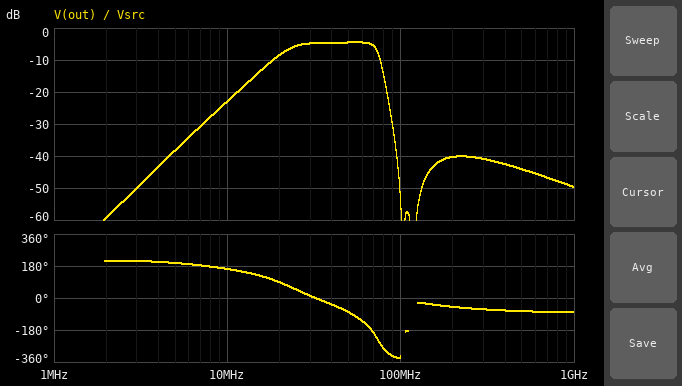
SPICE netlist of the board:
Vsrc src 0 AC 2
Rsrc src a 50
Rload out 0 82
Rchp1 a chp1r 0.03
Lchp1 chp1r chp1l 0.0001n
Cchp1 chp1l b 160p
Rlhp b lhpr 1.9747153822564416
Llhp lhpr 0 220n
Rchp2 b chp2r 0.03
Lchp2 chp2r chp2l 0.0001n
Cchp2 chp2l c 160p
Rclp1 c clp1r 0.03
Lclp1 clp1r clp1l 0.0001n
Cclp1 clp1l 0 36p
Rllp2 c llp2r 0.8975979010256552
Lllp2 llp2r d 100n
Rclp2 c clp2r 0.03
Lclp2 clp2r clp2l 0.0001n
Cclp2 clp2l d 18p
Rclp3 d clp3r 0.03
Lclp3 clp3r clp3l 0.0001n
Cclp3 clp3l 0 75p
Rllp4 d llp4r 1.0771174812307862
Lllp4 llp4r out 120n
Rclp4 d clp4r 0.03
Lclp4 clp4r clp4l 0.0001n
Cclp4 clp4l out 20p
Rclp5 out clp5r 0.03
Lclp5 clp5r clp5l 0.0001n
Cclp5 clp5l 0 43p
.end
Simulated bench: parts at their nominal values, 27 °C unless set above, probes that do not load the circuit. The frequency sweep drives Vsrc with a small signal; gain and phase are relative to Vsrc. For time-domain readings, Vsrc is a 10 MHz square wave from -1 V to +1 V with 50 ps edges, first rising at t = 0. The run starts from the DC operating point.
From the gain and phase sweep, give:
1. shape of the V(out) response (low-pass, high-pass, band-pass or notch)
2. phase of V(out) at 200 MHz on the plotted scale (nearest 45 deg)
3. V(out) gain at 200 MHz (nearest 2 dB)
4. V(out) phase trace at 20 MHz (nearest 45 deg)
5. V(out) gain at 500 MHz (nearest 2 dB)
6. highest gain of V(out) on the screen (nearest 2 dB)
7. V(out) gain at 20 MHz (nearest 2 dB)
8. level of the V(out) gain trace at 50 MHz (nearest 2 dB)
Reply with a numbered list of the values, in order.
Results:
1. band-pass
2. -45 deg
3. -40 dB
4. 90 deg
5. -44 dB
6. -4 dB
7. -8 dB
8. -4 dB
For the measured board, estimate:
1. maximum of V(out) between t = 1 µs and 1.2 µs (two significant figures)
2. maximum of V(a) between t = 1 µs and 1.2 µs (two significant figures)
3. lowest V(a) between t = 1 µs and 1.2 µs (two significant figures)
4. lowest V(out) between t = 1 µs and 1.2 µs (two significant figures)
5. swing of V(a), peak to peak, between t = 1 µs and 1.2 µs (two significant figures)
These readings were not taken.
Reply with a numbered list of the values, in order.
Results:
1. 490 mV
2. 1.2 V
3. -1.2 V
4. -490 mV
5. 2.4 V
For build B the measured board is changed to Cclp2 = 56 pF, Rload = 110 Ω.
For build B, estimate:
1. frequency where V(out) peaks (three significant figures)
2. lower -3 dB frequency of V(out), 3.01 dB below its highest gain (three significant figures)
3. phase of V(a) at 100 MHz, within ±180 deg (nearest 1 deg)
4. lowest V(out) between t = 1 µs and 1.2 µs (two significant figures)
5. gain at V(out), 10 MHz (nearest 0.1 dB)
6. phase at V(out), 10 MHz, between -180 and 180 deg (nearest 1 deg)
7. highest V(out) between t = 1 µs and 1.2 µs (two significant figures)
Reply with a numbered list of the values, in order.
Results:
1. 33.4 MHz
2. 21.4 MHz
3. -39 deg
4. -460 mV
5. -22.5 dB
6. 158 deg
7. 460 mV
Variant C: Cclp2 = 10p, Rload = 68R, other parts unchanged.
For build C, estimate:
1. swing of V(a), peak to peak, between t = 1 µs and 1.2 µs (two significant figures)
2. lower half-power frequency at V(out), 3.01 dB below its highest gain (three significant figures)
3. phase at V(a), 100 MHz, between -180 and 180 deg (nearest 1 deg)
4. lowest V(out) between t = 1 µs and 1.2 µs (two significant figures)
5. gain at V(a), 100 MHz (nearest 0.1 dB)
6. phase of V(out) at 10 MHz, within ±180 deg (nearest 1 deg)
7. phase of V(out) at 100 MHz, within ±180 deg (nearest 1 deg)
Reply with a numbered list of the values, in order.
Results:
1. 2.3 V
2. 20.7 MHz
3. -6 deg
4. -440 mV
5. -0.2 dB
6. 167 deg
7. 42 deg
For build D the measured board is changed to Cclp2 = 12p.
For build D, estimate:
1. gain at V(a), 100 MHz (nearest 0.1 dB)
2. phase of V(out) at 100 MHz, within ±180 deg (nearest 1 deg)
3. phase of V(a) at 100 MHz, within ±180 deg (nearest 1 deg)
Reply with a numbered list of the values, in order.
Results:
1. -0.3 dB
2. 33 deg
3. -10 deg
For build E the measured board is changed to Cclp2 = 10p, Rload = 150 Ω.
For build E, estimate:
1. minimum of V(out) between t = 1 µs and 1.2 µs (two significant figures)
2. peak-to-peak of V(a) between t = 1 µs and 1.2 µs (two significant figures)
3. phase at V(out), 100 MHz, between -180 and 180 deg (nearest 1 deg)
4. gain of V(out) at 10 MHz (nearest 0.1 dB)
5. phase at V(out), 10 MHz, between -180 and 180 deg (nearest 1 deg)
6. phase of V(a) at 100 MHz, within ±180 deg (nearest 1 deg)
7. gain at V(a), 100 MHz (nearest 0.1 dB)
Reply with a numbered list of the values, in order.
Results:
1. -570 mV
2. 2.5 V
3. 27 deg
4. -22.3 dB
5. 153 deg
6. -6 deg
7. -0.2 dB
